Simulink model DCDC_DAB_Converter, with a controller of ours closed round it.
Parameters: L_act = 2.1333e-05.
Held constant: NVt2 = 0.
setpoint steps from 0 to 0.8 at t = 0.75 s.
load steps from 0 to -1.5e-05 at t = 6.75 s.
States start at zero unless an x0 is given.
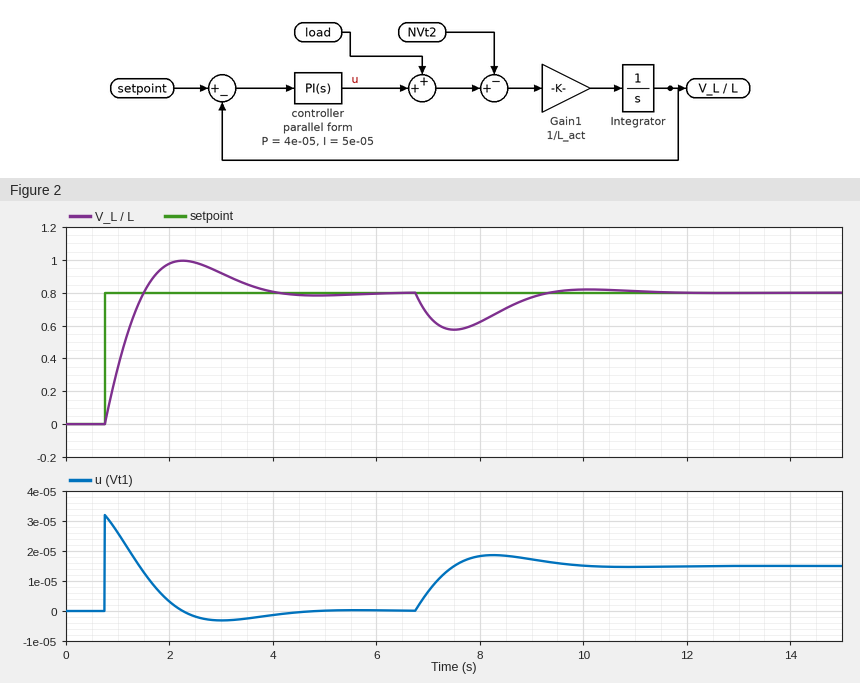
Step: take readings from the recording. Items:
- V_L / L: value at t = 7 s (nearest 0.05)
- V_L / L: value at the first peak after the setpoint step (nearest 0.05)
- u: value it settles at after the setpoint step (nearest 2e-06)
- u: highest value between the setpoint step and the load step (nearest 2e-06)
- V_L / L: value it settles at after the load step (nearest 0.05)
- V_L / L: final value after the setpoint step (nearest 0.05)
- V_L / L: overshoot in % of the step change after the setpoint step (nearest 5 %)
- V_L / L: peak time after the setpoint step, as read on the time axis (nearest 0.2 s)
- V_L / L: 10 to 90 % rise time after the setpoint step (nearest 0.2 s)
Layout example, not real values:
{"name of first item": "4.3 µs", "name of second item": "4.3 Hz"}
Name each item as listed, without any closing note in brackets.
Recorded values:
{"V_L / L: value at t = 7 s": "0.65", "V_L / L: value at the first peak after the setpoint step": "1.00", "u: value it settles at after the setpoint step": "0.000000", "u: highest value between the setpoint step and the load step": "0.000032", "V_L / L: value it settles at after the load step": "0.80", "V_L / L: final value after the setpoint step": "0.80", "V_L / L: overshoot in % of the step change after the setpoint step": "25 %", "V_L / L: peak time after the setpoint step, as read on the time axis": "2.2 s", "V_L / L: 10 to 90 % rise time after the setpoint step": "0.6 s"}
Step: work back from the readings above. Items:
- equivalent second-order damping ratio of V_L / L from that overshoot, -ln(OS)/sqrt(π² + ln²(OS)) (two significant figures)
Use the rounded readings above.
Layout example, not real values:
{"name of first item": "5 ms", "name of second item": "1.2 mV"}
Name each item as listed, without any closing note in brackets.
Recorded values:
{"equivalent second-order damping ratio of V_L / L from that overshoot, -ln(OS)/sqrt(π² + ln²(OS))": "0.40"}
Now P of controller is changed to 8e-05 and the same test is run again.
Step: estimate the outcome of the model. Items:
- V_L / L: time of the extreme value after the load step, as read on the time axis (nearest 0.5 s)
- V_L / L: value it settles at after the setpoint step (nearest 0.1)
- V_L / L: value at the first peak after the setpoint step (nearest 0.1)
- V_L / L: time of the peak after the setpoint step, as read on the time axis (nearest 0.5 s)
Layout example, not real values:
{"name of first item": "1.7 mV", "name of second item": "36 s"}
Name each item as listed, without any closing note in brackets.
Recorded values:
{"V_L / L: time of the extreme value after the load step, as read on the time axis": "7.5 s", "V_L / L: value it settles at after the setpoint step": "0.8", "V_L / L: value at the first peak after the setpoint step": "0.9", "V_L / L: time of the peak after the setpoint step, as read on the time axis": "2.0 s"}
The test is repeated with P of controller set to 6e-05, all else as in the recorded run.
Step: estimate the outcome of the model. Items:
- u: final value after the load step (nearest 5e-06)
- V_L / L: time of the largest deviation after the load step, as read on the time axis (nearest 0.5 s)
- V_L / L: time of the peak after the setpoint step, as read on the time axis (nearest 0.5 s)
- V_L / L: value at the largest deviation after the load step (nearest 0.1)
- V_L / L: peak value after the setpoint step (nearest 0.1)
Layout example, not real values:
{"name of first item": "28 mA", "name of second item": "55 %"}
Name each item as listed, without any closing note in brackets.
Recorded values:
{"u: final value after the load step": "0.000015", "V_L / L: time of the largest deviation after the load step, as read on the time axis": "7.5 s", "V_L / L: time of the peak after the setpoint step, as read on the time axis": "2.0 s", "V_L / L: value at the largest deviation after the load step": "0.6", "V_L / L: peak value after the setpoint step": "0.9"}
